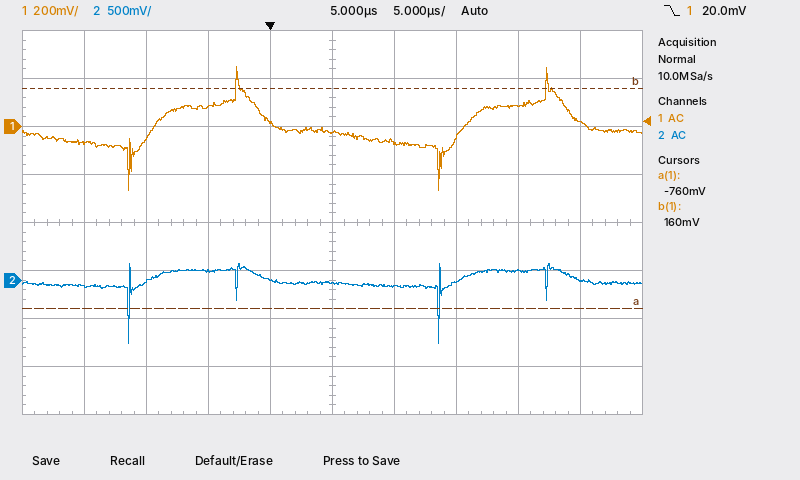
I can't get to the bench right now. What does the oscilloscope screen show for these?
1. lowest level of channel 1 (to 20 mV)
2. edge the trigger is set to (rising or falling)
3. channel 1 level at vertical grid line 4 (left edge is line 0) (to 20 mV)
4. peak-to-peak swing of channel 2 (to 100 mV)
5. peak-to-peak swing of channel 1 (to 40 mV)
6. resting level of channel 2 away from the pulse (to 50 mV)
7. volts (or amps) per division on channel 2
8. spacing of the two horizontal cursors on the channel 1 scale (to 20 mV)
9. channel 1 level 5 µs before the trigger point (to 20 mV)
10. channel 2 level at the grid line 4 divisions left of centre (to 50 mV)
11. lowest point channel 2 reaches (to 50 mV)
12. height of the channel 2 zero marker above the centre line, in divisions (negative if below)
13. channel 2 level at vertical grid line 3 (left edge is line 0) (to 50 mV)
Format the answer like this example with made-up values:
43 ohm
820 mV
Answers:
-260 mV
falling
20 mV
800 mV
520 mV
-50 mV
500 mV
920 mV
80 mV
-50 mV
-650 mV
-1.2 div
100 mV
